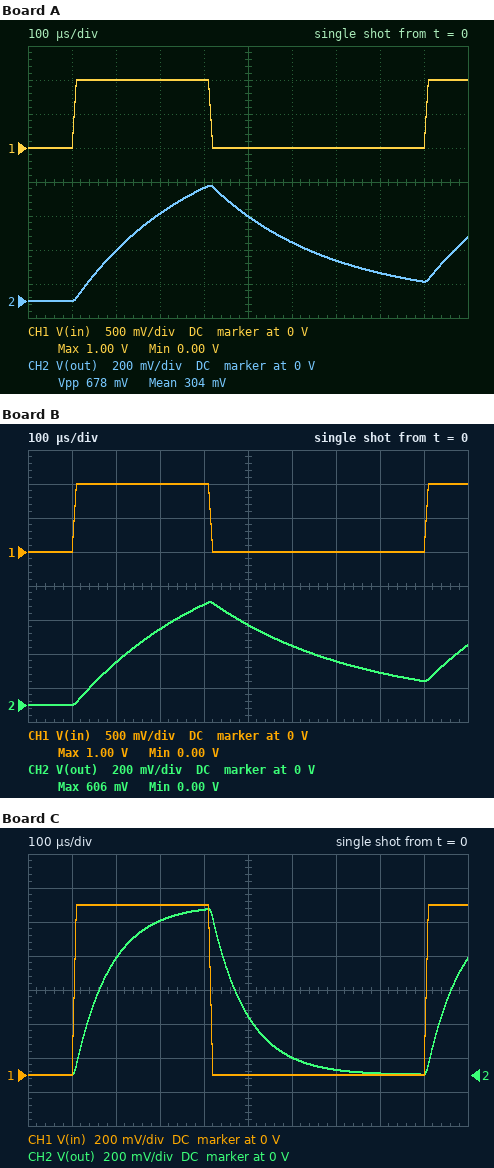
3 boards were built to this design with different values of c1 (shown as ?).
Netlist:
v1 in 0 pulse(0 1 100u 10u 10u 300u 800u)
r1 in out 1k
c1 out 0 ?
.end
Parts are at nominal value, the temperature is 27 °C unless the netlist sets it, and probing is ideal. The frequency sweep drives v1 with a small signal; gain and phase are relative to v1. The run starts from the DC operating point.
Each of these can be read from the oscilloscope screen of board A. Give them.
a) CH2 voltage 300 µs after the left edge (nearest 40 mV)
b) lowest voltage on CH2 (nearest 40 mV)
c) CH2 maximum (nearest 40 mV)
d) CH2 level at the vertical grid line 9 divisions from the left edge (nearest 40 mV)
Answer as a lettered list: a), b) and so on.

a) 520 mV
b) 0 V
c) 680 mV
d) 120 mV
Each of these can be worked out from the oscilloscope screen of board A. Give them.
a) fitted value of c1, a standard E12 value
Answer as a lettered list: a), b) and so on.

a) 270 nF
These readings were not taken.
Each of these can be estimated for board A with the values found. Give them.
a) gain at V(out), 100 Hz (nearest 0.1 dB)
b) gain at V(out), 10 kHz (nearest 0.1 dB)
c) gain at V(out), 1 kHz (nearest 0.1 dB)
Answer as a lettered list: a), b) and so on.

a) -0.1 dB
b) -24.6 dB
c) -5.9 dB
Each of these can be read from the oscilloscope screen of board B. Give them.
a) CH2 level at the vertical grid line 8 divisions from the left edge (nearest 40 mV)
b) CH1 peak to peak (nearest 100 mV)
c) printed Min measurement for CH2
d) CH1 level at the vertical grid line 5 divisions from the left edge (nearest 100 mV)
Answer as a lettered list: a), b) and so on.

a) 200 mV
b) 1.0 V
c) 0.00 V
d) 0 V
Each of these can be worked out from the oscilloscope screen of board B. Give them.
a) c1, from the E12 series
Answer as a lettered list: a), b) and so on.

a) 330 nF
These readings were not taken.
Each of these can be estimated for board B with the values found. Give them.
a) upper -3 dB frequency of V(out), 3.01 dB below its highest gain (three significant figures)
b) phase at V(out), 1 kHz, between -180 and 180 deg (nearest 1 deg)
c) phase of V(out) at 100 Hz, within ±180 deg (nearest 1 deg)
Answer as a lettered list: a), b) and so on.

a) 482 Hz
b) -64 deg
c) -12 deg
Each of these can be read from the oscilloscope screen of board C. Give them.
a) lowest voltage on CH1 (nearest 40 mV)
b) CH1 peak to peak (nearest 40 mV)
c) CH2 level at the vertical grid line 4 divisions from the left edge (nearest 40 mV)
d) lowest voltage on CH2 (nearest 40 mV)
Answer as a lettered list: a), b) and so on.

a) 0 V
b) 1.00 V
c) 960 mV
d) 0 V
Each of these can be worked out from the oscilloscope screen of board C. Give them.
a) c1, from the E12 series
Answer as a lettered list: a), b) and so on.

a) 82 nF
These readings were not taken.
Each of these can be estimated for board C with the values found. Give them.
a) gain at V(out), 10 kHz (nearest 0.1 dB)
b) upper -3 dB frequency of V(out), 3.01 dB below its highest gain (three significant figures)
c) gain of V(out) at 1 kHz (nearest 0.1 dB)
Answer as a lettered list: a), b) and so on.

a) -14.4 dB
b) 1.94 kHz
c) -1.0 dB
